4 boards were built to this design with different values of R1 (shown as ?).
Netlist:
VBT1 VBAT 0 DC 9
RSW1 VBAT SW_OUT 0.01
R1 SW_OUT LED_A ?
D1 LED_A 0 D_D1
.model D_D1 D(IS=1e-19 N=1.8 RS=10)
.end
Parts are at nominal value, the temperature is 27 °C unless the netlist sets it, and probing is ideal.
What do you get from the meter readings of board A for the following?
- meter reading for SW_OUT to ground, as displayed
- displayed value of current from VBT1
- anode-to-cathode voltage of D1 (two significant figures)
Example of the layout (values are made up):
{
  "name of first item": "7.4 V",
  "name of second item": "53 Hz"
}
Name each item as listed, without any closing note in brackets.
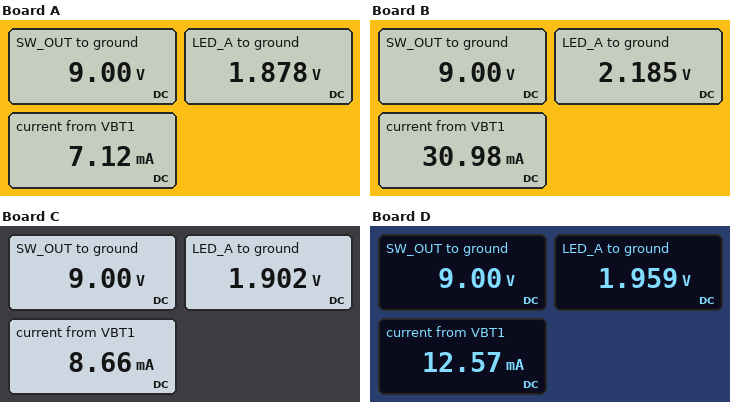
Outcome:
{
  "meter reading for SW_OUT to ground, as displayed": "9.00 V",
  "displayed value of current from VBT1": "7.12 mA",
  "anode-to-cathode voltage of D1": "1.9 V"
}
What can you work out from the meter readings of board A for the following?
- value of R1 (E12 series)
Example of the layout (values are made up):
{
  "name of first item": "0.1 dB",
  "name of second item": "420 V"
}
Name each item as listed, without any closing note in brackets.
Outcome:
{
  "value of R1": "1 kΩ"
}
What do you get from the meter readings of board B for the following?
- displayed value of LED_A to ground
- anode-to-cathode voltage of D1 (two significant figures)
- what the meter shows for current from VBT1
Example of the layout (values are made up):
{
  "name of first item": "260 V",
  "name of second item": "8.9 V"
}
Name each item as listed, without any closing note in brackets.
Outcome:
{
  "displayed value of LED_A to ground": "2.185 V",
  "anode-to-cathode voltage of D1": "2.2 V",
  "what the meter shows for current from VBT1": "30.98 mA"
}
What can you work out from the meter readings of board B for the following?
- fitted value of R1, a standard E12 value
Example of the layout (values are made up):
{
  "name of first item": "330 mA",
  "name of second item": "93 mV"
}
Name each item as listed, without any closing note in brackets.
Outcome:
{
  "fitted value of R1, a standard E12 value": "220 Ω"
}
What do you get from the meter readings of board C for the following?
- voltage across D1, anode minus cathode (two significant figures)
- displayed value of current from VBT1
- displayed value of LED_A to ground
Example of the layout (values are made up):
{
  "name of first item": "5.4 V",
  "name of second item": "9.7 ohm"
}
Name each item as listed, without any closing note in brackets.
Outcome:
{
  "voltage across D1, anode minus cathode": "1.9 V",
  "displayed value of current from VBT1": "8.66 mA",
  "displayed value of LED_A to ground": "1.902 V"
}
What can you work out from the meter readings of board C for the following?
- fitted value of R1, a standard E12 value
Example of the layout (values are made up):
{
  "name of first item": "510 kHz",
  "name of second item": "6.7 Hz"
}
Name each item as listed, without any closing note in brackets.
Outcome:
{
  "fitted value of R1, a standard E12 value": "820 Ω"
}
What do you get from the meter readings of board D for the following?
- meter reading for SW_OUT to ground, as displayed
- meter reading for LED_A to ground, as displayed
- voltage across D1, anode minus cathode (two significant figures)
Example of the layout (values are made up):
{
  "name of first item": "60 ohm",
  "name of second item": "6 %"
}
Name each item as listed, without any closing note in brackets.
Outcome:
{
  "meter reading for SW_OUT to ground, as displayed": "9.00 V",
  "meter reading for LED_A to ground, as displayed": "1.959 V",
  "voltage across D1, anode minus cathode": "2.0 V"
}
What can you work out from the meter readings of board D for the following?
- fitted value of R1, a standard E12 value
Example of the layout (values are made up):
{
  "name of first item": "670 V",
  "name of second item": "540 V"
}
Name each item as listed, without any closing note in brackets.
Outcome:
{
  "fitted value of R1, a standard E12 value": "560 Ω"
}
